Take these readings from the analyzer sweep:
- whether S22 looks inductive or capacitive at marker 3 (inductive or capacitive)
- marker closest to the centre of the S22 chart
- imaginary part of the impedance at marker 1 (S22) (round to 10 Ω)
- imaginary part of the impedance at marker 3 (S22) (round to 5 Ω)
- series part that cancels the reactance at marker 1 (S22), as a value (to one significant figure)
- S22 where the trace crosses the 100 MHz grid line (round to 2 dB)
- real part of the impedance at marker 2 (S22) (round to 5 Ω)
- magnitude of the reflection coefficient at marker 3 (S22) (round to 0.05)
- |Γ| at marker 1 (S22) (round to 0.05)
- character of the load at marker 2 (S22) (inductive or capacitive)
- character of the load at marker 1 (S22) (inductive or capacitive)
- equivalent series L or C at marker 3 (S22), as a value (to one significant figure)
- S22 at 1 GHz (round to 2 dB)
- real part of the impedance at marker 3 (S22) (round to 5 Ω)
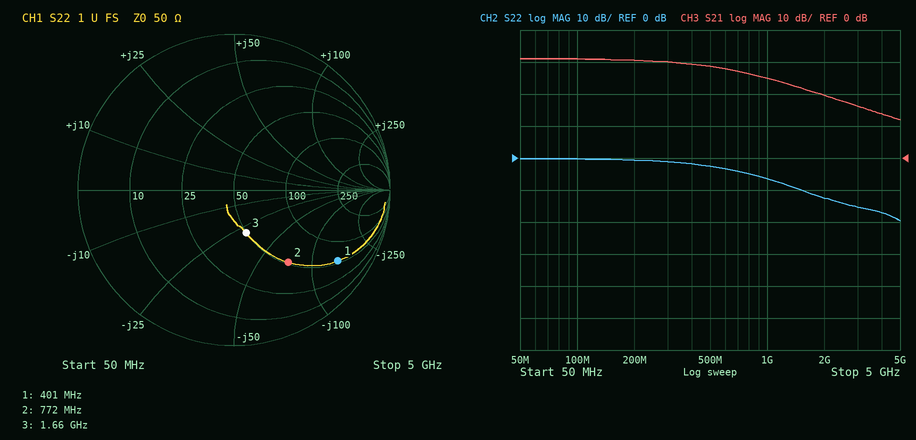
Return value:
capacitive
marker 3
-140 Ω
-30 Ω
60 nH
0 dB
50 Ω
0.30
0.80
capacitive
capacitive
3 pF
-6 dB
50 Ω
